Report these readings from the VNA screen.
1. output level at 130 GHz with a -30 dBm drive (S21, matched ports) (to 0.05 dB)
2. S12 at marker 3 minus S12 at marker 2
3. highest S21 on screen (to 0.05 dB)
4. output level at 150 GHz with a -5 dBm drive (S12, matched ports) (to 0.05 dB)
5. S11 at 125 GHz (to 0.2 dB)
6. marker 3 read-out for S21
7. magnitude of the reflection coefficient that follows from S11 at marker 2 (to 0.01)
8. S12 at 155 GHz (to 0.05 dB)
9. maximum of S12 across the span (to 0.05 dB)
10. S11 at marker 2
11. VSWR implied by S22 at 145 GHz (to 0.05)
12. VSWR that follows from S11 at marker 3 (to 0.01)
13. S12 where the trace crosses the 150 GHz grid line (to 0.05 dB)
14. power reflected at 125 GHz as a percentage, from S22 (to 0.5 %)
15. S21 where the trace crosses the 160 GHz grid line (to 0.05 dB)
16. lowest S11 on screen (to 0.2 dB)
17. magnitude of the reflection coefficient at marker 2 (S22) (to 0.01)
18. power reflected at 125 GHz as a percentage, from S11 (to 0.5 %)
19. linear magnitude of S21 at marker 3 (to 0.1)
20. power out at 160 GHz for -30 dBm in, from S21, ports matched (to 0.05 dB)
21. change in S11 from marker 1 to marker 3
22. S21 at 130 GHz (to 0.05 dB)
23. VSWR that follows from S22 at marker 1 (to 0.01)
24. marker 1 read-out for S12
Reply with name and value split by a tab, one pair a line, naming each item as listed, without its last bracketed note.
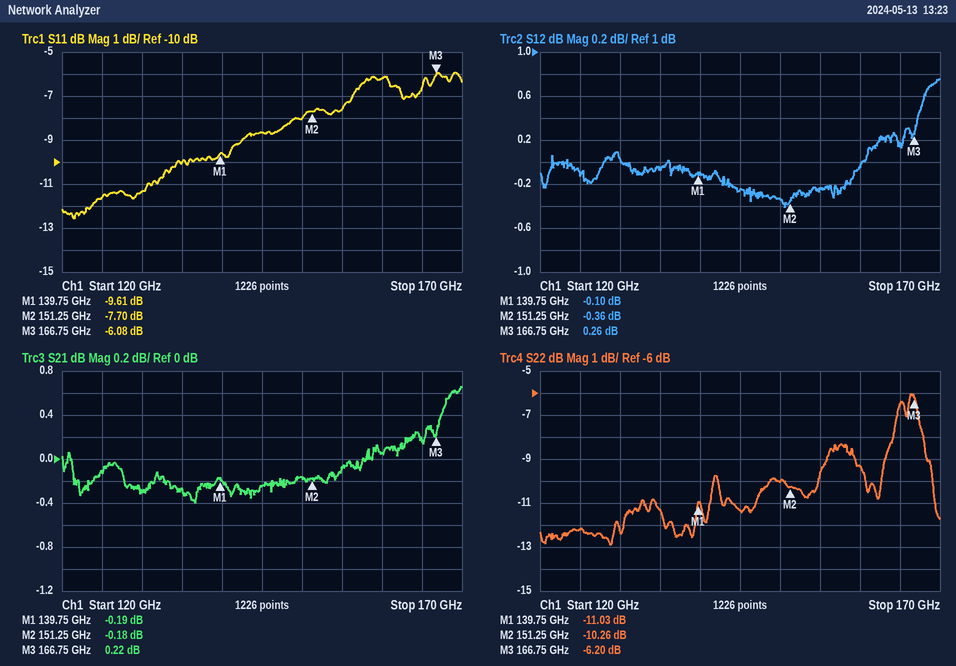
output level at 130 GHz with a -30 dBm drive (S21, matched ports)	-30.30 dBm
S12 at marker 3 minus S12 at marker 2	0.62 dB
highest S21 on screen	0.65 dB
output level at 150 GHz with a -5 dBm drive (S12, matched ports)	-5.35 dBm
S11 at 125 GHz	-11.6 dB
marker 3 read-out for S21	0.22 dB
magnitude of the reflection coefficient that follows from S11 at marker 2	0.41
S12 at 155 GHz	-0.25 dB
maximum of S12 across the span	0.75 dB
S11 at marker 2	-7.70 dB
VSWR implied by S22 at 145 GHz	1.75
VSWR that follows from S11 at marker 3	2.97
S12 where the trace crosses the 150 GHz grid line	-0.35 dB
power reflected at 125 GHz as a percentage, from S22	6.0 %
S21 where the trace crosses the 160 GHz grid line	0.05 dB
lowest S11 on screen	-12.6 dB
magnitude of the reflection coefficient at marker 2 (S22)	0.31
power reflected at 125 GHz as a percentage, from S11	7.0 %
linear magnitude of S21 at marker 3	1.0
power out at 160 GHz for -30 dBm in, from S21, ports matched	-29.95 dBm
change in S11 from marker 1 to marker 3	3.53 dB
S21 at 130 GHz	-0.30 dB
VSWR that follows from S22 at marker 1	1.78
marker 1 read-out for S12	-0.10 dB
